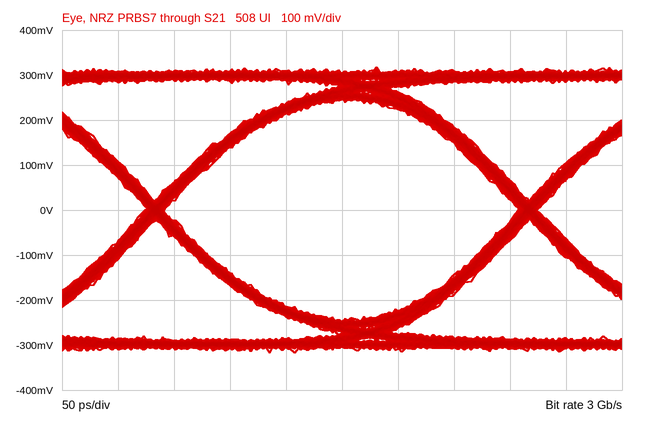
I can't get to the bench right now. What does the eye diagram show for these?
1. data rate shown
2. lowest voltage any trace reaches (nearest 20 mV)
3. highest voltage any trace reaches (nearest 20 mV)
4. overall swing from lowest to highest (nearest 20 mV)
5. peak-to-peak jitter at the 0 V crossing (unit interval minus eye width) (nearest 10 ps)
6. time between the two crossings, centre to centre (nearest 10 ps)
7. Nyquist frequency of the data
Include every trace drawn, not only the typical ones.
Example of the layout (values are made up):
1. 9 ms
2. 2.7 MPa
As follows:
1. 3 Gb/s
2. -320 mV
3. 320 mV
4. 640 mV
5. 20 ps
6. 330 ps
7. 1.5 GHz
